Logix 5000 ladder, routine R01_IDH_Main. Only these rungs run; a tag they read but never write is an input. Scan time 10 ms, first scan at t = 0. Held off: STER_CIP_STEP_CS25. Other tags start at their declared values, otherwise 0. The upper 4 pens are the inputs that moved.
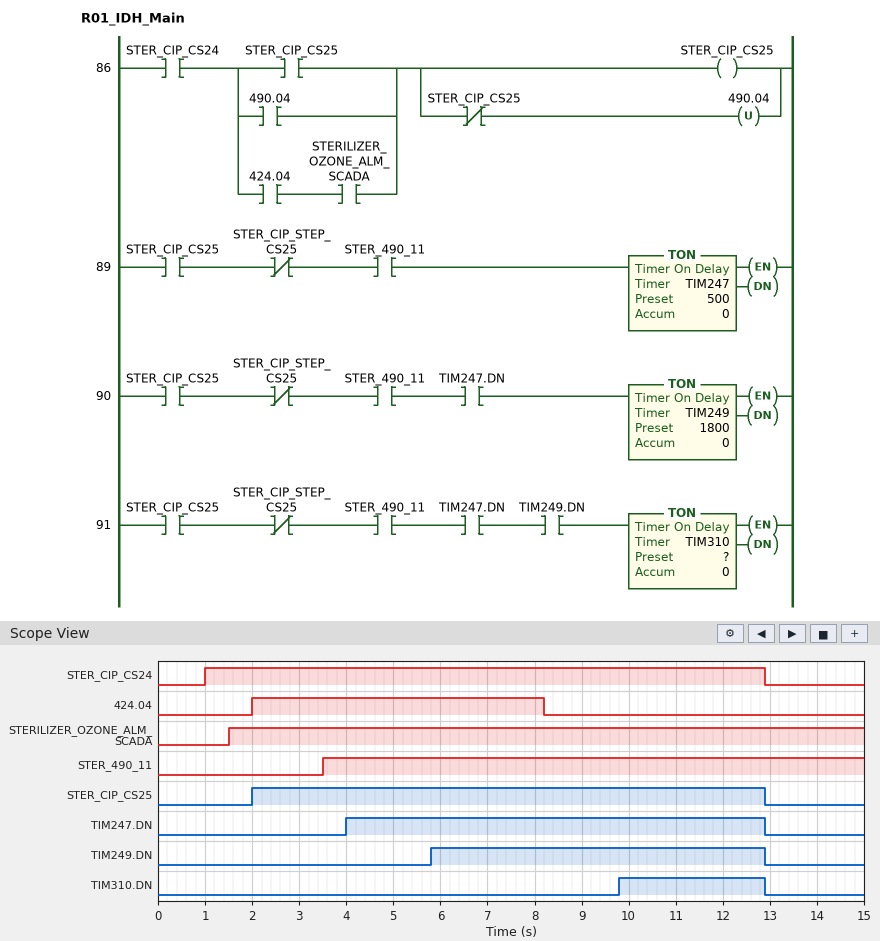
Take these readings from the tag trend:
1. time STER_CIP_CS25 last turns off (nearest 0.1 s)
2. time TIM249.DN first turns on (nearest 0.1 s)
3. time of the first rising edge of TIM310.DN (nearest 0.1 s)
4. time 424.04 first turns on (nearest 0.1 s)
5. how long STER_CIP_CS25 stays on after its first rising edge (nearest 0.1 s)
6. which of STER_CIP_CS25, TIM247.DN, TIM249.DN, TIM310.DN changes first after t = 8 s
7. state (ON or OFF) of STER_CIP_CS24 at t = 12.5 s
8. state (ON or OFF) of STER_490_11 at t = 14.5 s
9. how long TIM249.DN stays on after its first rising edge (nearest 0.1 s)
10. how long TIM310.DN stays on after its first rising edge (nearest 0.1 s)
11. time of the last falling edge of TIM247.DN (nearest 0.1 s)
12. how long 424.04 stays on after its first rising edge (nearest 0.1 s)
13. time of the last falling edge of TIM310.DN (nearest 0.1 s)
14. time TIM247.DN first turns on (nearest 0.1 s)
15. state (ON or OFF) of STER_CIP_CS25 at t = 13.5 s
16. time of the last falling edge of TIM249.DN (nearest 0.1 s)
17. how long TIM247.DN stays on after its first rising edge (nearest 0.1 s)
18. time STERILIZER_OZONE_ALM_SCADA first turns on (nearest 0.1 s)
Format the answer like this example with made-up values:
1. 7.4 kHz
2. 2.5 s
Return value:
1. 12.9 s
2. 5.8 s
3. 9.8 s
4. 2.0 s
5. 10.9 s
6. TIM310.DN
7. ON
8. ON
9. 7.1 s
10. 3.1 s
11. 12.9 s
12. 6.2 s
13. 12.9 s
14. 4.0 s
15. OFF
16. 12.9 s
17. 8.9 s
18. 1.5 s
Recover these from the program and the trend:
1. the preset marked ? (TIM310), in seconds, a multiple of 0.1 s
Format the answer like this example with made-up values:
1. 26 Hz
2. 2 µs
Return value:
1. 4.0 s
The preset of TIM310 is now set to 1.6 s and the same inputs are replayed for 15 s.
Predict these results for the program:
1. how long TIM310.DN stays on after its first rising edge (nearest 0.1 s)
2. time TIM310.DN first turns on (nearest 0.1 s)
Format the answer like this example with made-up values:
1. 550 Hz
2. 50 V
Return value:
1. 5.5 s
2. 7.4 s
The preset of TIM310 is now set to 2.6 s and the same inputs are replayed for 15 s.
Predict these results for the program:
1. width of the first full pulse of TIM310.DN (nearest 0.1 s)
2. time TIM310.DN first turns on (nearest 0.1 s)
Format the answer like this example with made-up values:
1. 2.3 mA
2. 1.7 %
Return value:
1. 4.5 s
2. 8.4 s
